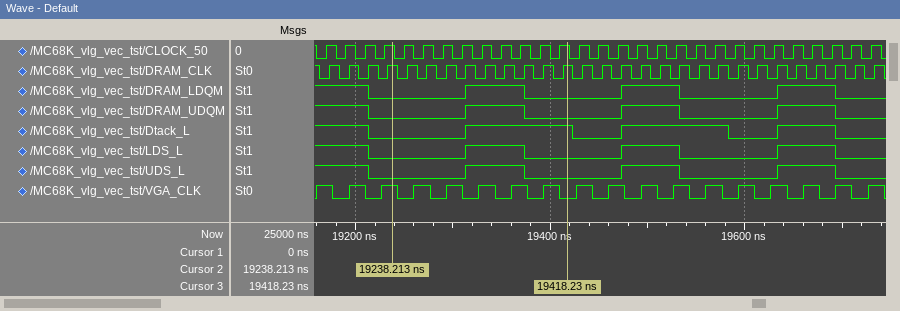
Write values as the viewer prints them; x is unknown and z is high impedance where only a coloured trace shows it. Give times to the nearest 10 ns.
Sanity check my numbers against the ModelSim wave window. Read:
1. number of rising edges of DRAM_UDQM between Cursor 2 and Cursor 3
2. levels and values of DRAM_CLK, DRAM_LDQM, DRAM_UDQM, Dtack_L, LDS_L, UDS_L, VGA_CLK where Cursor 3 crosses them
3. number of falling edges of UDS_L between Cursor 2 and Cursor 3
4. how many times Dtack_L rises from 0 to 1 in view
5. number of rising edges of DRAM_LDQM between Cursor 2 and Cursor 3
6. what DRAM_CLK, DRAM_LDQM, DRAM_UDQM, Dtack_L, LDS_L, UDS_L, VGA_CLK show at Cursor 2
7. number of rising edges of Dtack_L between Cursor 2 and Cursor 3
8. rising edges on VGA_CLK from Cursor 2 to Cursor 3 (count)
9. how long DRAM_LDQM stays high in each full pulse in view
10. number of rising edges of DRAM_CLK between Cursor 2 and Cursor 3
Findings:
1
DRAM_CLK=1, DRAM_LDQM=0, DRAM_UDQM=0, Dtack_L=1, LDS_L=0, UDS_L=0, VGA_CLK=0
1
3
1
DRAM_CLK=1, DRAM_LDQM=0, DRAM_UDQM=0, Dtack_L=0, LDS_L=0, UDS_L=0, VGA_CLK=1
1
5
60 ns, 60 ns, 60 ns
9
